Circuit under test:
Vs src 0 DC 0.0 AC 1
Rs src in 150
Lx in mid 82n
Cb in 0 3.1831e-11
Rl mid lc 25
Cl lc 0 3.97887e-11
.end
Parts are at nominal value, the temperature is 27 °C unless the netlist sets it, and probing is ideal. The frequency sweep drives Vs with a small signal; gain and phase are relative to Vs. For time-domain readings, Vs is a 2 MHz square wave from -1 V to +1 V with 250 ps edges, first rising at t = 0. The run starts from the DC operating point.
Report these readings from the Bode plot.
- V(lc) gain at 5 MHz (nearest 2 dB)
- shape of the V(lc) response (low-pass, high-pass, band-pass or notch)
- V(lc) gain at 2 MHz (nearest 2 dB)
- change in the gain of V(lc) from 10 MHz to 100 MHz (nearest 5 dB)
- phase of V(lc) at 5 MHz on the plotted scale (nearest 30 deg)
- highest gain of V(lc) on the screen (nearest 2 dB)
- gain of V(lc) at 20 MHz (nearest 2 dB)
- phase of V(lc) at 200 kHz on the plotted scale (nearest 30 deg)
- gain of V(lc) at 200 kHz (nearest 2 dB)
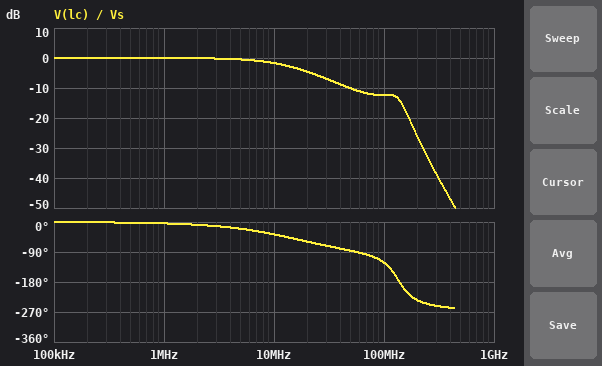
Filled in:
0 dB
low-pass
0 dB
-10 dB
-30 deg
0 dB
-4 dB
0 deg
0 dB
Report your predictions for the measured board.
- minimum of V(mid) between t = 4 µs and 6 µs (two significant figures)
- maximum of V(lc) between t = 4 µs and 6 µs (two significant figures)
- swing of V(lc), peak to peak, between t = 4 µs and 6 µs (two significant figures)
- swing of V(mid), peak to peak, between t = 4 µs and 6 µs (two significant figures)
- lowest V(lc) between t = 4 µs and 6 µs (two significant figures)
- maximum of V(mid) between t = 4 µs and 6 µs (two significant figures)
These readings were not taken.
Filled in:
-1.0 V
1.0 V
2.0 V
2.0 V
-1.0 V
1.0 V
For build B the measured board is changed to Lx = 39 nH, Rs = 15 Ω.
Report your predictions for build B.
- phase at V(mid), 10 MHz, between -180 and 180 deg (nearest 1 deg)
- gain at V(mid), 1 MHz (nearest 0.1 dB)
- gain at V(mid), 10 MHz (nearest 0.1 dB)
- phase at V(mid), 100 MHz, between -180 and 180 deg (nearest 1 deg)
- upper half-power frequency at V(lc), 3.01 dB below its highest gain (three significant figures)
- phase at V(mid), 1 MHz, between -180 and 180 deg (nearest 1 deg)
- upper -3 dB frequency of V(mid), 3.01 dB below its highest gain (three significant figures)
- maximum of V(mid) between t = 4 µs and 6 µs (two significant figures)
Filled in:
-4 deg
0 dB
0 dB
-48 deg
138 MHz
0 deg
179 MHz
1.2 V
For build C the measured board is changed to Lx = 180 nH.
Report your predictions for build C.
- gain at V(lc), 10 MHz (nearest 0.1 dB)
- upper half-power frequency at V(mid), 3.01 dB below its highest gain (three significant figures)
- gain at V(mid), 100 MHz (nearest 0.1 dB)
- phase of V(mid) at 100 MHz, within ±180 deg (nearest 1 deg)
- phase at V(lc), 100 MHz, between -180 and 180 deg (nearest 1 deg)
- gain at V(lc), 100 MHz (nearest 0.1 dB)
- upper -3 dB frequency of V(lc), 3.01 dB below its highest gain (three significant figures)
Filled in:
-1.6 dB
15.5 MHz
-10.3 dB
-165 deg
163 deg
-11.7 dB
15.3 MHz
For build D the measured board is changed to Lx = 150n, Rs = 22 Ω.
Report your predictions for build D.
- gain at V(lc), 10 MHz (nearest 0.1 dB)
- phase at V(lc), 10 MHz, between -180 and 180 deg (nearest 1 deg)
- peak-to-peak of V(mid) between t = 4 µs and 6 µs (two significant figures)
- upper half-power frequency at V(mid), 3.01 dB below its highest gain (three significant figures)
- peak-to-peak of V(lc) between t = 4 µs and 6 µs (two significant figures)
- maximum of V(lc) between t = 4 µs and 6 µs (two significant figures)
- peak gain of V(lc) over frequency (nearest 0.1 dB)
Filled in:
0.1 dB
-9 deg
3.1 V
83.3 MHz
3.0 V
1.5 V
2.6 dB
